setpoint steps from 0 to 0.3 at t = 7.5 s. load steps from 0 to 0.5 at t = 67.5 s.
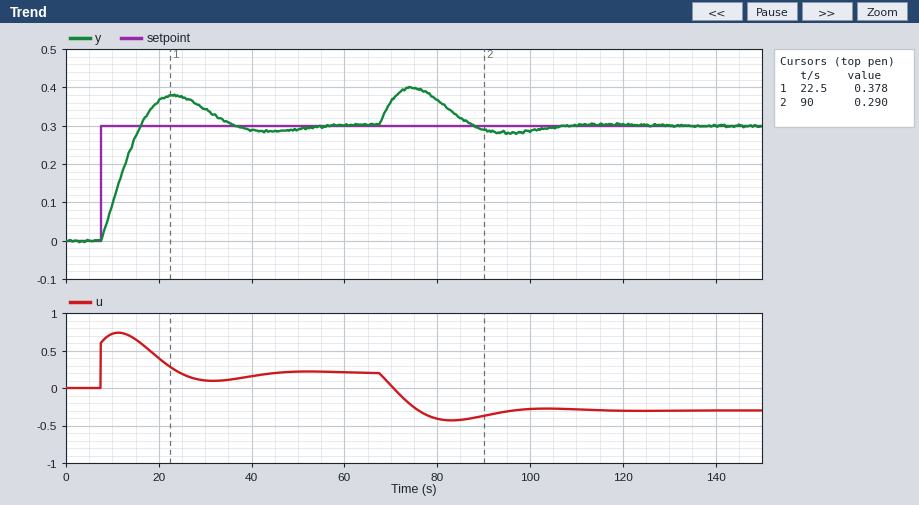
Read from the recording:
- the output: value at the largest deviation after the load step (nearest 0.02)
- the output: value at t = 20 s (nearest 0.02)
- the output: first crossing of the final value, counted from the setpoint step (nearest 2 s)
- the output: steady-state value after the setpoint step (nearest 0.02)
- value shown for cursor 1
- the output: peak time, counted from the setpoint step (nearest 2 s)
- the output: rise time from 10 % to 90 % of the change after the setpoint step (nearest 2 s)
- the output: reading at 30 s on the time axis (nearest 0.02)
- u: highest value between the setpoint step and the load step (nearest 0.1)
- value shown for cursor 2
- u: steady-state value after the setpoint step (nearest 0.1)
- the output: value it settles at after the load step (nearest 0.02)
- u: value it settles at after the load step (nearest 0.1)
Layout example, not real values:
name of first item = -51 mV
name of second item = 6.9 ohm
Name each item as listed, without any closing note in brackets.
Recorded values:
the output: value at the largest deviation after the load step = 0.40
the output: value at t = 20 s = 0.36
the output: first crossing of the final value, counted from the setpoint step = 8 s
the output: steady-state value after the setpoint step = 0.30
value shown for cursor 1 = 0.378
the output: peak time, counted from the setpoint step = 16 s
the output: rise time from 10 % to 90 % of the change after the setpoint step = 6 s
the output: reading at 30 s on the time axis = 0.34
u: highest value between the setpoint step and the load step = 0.7
value shown for cursor 2 = 0.290
u: steady-state value after the setpoint step = 0.2
the output: value it settles at after the load step = 0.30
u: value it settles at after the load step = -0.3
